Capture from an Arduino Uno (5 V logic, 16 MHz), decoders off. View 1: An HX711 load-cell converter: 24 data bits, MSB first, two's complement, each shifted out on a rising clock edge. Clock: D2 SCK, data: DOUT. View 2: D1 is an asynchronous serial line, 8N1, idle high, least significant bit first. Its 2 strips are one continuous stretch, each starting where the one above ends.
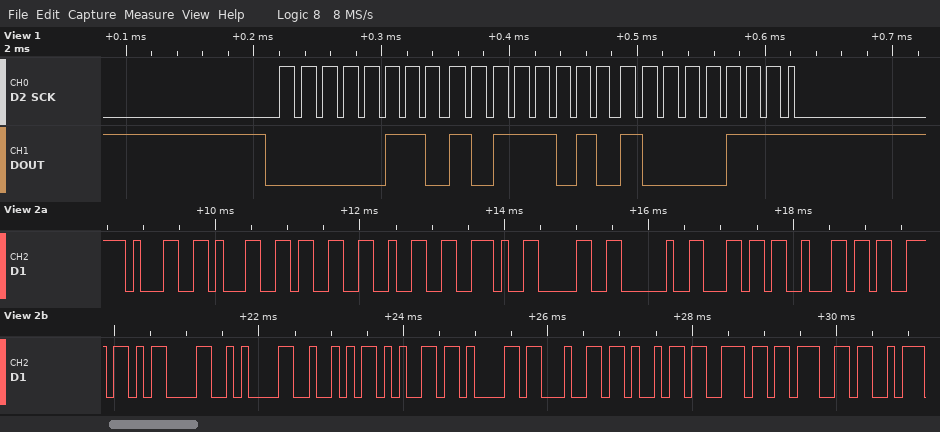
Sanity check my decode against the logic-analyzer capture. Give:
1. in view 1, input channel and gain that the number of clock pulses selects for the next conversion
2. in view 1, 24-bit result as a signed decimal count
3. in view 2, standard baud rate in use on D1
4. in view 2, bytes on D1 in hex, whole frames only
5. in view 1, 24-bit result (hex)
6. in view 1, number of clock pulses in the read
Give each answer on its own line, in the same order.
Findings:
channel A, gain 128
440967
9600 baud
31 31 33 32 2E 30 20 6C 62 73 0D 0A 52 65 61 64 69 6E 67
0x06BA87
25
